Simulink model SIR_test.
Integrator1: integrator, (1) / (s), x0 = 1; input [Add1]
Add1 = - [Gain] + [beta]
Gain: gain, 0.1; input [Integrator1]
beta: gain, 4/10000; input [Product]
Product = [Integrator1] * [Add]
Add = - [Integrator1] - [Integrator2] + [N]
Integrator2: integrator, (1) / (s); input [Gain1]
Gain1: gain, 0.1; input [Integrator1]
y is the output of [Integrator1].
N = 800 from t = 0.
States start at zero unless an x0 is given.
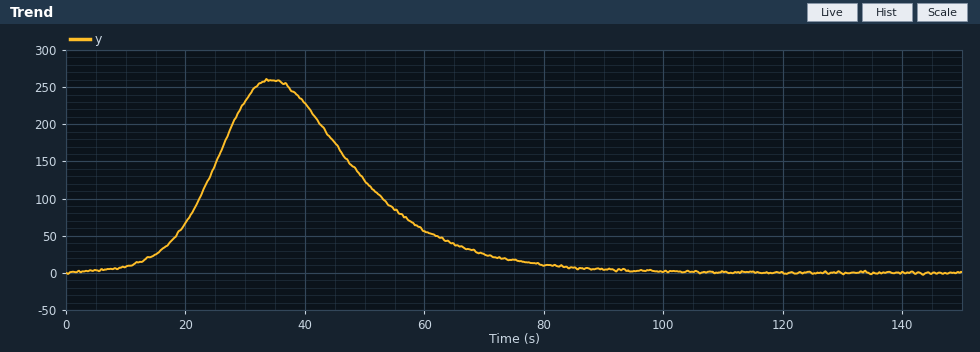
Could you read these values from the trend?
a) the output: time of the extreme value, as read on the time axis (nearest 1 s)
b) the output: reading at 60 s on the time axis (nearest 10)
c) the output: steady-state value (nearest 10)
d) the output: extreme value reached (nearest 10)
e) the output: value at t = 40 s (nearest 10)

34 s
60
0
260
230
